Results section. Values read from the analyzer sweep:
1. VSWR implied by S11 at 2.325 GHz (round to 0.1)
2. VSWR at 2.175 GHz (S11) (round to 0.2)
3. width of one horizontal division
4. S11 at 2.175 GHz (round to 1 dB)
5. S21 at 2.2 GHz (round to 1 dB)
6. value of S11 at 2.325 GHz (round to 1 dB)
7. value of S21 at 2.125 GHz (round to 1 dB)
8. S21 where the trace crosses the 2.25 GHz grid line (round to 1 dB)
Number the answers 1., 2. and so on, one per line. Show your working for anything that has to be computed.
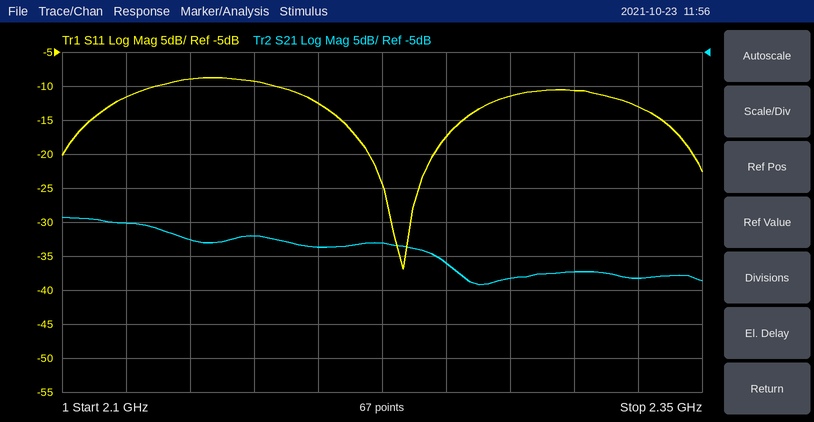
1. |Γ| = 10^(-13/20) = 0.2239; VSWR = (1 + 0.2239)/(1 − 0.2239) ≈ 1.6
2. |Γ| = 10^(-9/20) = 0.3548; VSWR = (1 + 0.3548)/(1 − 0.3548) ≈ 2.10, so 2.0 to the nearest 0.2
3. 25 MHz
4. -9 dB
5. -34 dB
6. -13 dB
7. -30 dB
8. -36 dB
